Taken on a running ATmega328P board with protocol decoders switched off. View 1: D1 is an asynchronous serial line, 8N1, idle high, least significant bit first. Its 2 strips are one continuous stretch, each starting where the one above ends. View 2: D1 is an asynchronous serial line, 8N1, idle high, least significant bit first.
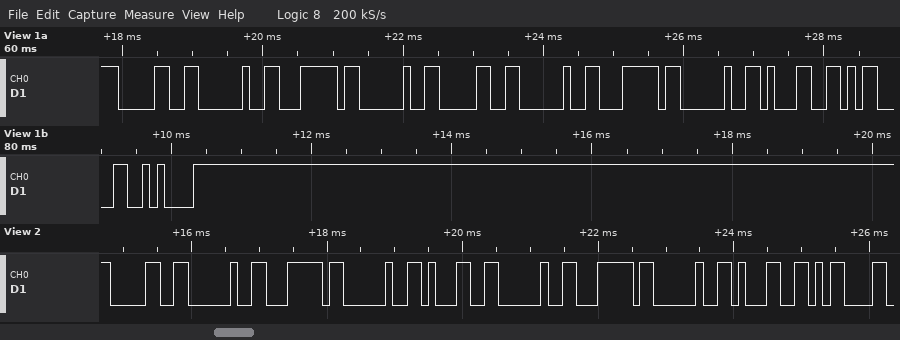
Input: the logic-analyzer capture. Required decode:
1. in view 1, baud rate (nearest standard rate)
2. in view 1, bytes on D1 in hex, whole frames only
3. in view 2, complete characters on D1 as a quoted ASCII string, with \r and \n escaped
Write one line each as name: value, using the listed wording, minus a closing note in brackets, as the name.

in view 1, baud rate: 9600 baud
in view 1, bytes on D1 in hex, whole frames only: 0x30 0x20 0x7C 0x20 0x30 0x20 0x7C 0x20 0x31 0x0D 0x0A
in view 2, complete characters on D1 as a quoted ASCII string, with \r and \n escaped: "0 | 1 | 1\r"
